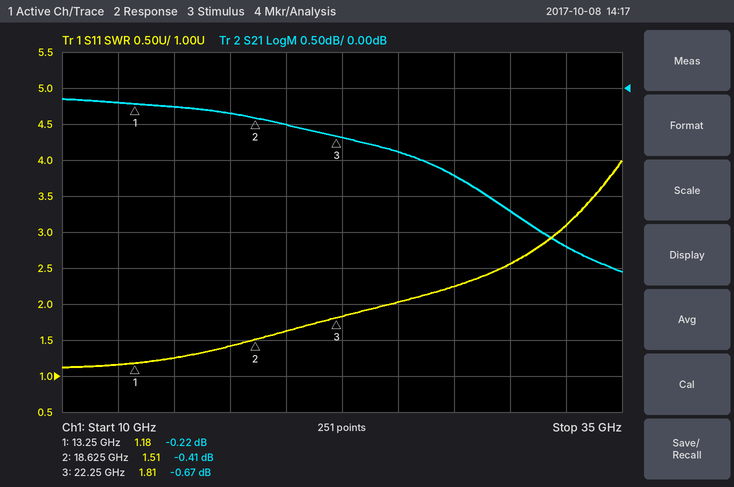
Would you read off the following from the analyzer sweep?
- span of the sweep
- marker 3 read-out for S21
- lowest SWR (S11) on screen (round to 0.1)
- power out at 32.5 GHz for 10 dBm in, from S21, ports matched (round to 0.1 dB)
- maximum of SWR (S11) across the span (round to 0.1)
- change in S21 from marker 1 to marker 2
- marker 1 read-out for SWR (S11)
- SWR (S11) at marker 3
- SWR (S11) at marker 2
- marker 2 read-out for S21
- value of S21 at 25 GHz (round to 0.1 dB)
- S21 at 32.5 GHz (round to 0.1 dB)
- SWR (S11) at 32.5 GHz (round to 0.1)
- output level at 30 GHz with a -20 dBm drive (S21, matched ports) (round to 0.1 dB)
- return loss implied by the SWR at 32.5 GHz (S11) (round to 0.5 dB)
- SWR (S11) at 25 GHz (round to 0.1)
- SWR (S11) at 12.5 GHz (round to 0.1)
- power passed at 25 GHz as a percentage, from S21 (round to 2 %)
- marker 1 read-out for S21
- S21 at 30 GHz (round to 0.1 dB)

25 GHz
-0.67 dB
1.1
7.8 dBm
4.0
-0.19 dB
1.18
1.81
1.51
-0.41 dB
-0.9 dB
-2.2 dB
3.1
-21.7 dBm
6.0 dB
2.0
1.2
82 %
-0.22 dB
-1.7 dB
